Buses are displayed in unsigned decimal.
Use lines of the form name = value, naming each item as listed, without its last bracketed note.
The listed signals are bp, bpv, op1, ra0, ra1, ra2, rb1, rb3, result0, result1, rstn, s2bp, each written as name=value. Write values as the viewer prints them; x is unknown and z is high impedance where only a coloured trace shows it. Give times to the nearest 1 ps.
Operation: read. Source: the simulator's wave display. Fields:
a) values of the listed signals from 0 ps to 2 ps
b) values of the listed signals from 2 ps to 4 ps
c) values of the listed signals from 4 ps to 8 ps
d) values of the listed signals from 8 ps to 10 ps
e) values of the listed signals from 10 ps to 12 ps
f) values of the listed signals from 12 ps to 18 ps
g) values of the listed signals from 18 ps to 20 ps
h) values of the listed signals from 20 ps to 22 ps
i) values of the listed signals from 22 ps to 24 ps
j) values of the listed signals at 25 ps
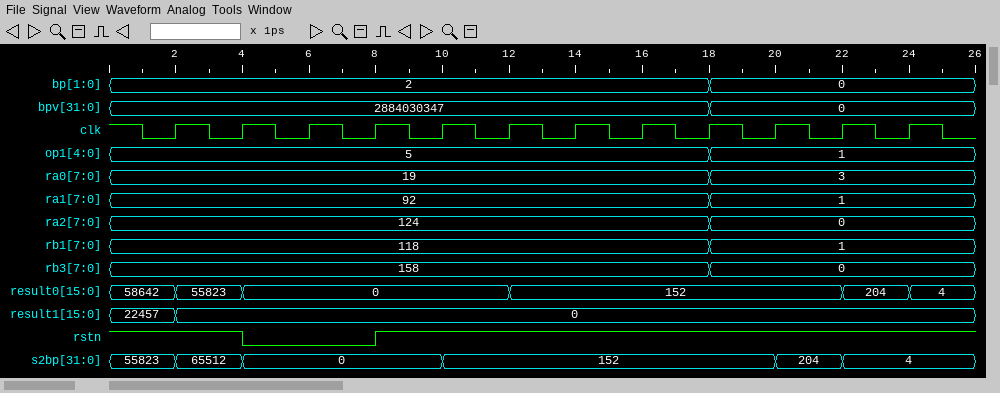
values of the listed signals from 0 ps to 2 ps = bp=2, bpv=2884030347, op1=5, ra0=19, ra1=92, ra2=124, rb1=118, rb3=158, result0=58642, result1=22457, rstn=1, s2bp=55823
values of the listed signals from 2 ps to 4 ps = bp=2, bpv=2884030347, op1=5, ra0=19, ra1=92, ra2=124, rb1=118, rb3=158, result0=55823, result1=0, rstn=1, s2bp=65512
values of the listed signals from 4 ps to 8 ps = bp=2, bpv=2884030347, op1=5, ra0=19, ra1=92, ra2=124, rb1=118, rb3=158, result0=0, result1=0, rstn=0, s2bp=0
values of the listed signals from 8 ps to 10 ps = bp=2, bpv=2884030347, op1=5, ra0=19, ra1=92, ra2=124, rb1=118, rb3=158, result0=0, result1=0, rstn=1, s2bp=0
values of the listed signals from 10 ps to 12 ps = bp=2, bpv=2884030347, op1=5, ra0=19, ra1=92, ra2=124, rb1=118, rb3=158, result0=0, result1=0, rstn=1, s2bp=152
values of the listed signals from 12 ps to 18 ps = bp=2, bpv=2884030347, op1=5, ra0=19, ra1=92, ra2=124, rb1=118, rb3=158, result0=152, result1=0, rstn=1, s2bp=152
values of the listed signals from 18 ps to 20 ps = bp=0, bpv=0, op1=1, ra0=3, ra1=1, ra2=0, rb1=1, rb3=0, result0=152, result1=0, rstn=1, s2bp=152
values of the listed signals from 20 ps to 22 ps = bp=0, bpv=0, op1=1, ra0=3, ra1=1, ra2=0, rb1=1, rb3=0, result0=152, result1=0, rstn=1, s2bp=204
values of the listed signals from 22 ps to 24 ps = bp=0, bpv=0, op1=1, ra0=3, ra1=1, ra2=0, rb1=1, rb3=0, result0=204, result1=0, rstn=1, s2bp=4
values of the listed signals at 25 ps = bp=0, bpv=0, op1=1, ra0=3, ra1=1, ra2=0, rb1=1, rb3=0, result0=4, result1=0, rstn=1, s2bp=4
